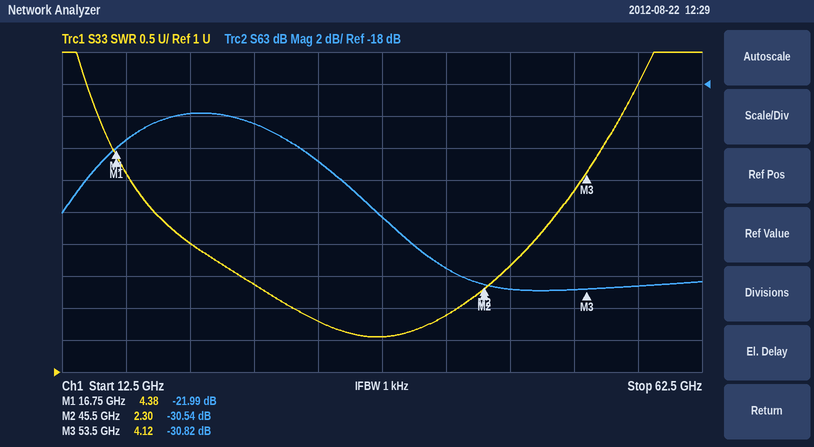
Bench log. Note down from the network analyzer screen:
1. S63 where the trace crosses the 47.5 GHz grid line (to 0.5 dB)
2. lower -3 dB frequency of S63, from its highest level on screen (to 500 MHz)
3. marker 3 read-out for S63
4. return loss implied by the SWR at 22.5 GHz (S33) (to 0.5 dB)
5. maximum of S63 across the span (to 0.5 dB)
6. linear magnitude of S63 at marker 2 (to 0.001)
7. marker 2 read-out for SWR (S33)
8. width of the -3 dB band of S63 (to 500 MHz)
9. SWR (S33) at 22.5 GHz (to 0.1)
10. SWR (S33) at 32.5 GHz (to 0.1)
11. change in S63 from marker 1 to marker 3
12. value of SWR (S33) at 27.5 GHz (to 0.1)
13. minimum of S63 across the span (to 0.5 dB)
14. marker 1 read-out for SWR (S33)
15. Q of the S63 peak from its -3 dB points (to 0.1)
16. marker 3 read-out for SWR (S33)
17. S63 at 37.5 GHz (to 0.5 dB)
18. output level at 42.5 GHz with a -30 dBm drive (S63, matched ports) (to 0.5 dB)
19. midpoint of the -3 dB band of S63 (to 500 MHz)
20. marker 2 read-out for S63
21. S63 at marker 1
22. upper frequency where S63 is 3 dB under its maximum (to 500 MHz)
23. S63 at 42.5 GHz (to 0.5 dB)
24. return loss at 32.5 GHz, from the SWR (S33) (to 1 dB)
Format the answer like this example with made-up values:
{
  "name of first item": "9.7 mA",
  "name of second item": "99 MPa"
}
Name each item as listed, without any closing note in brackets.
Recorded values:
{
  "S63 where the trace crosses the 47.5 GHz grid line": "-31.0 dB",
  "lower -3 dB frequency of S63, from its highest level on screen": "15.5 GHz",
  "marker 3 read-out for S63": "-30.82 dB",
  "return loss implied by the SWR at 22.5 GHz (S33)": "6.0 dB",
  "maximum of S63 across the span": "-20.0 dB",
  "linear magnitude of S63 at marker 2": "0.030",
  "marker 2 read-out for SWR": "2.30",
  "width of the -3 dB band of S63": "17.0 GHz",
  "SWR (S33) at 22.5 GHz": "3.0",
  "SWR (S33) at 32.5 GHz": "1.8",
  "change in S63 from marker 1 to marker 3": "-8.83 dB",
  "value of SWR (S33) at 27.5 GHz": "2.4",
  "minimum of S63 across the span": "-31.0 dB",
  "marker 1 read-out for SWR": "4.38",
  "Q of the S63 peak from its -3 dB points": "1.4",
  "marker 3 read-out for SWR": "4.12",
  "S63 at 37.5 GHz": "-26.5 dB",
  "output level at 42.5 GHz with a -30 dBm drive (S63, matched ports)": "-59.5 dBm",
  "midpoint of the -3 dB band of S63": "24.0 GHz",
  "marker 2 read-out for S63": "-30.54 dB",
  "S63 at marker 1": "-21.99 dB",
  "upper frequency where S63 is 3 dB under its maximum": "32.5 GHz",
  "S63 at 42.5 GHz": "-29.5 dB",
  "return loss at 32.5 GHz, from the SWR (S33)": "11 dB"
}
